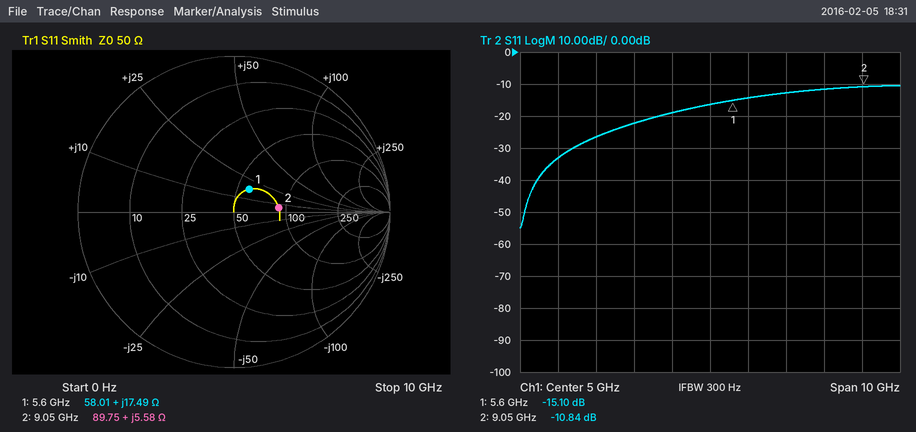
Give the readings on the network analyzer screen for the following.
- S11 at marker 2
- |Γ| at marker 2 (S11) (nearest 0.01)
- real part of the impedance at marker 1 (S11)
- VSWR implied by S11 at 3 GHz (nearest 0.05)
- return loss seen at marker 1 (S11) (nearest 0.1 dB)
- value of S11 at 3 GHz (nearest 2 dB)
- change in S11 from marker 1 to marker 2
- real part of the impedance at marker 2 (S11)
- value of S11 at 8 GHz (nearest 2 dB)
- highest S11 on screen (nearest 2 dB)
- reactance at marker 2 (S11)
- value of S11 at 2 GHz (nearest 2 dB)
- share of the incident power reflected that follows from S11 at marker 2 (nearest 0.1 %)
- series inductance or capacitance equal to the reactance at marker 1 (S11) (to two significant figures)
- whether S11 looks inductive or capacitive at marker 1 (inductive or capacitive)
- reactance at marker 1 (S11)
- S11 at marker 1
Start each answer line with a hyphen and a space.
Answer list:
- -10.84 dB
- 0.29
- 58.01 Ω
- 1.15
- 15.1 dB
- -22 dB
- 4.26 dB
- 89.75 Ω
- -12 dB
- -10 dB
- +5.58 Ω
- -26 dB
- 8.2 %
- 500 pH
- inductive
- +17.49 Ω
- -15.10 dB
